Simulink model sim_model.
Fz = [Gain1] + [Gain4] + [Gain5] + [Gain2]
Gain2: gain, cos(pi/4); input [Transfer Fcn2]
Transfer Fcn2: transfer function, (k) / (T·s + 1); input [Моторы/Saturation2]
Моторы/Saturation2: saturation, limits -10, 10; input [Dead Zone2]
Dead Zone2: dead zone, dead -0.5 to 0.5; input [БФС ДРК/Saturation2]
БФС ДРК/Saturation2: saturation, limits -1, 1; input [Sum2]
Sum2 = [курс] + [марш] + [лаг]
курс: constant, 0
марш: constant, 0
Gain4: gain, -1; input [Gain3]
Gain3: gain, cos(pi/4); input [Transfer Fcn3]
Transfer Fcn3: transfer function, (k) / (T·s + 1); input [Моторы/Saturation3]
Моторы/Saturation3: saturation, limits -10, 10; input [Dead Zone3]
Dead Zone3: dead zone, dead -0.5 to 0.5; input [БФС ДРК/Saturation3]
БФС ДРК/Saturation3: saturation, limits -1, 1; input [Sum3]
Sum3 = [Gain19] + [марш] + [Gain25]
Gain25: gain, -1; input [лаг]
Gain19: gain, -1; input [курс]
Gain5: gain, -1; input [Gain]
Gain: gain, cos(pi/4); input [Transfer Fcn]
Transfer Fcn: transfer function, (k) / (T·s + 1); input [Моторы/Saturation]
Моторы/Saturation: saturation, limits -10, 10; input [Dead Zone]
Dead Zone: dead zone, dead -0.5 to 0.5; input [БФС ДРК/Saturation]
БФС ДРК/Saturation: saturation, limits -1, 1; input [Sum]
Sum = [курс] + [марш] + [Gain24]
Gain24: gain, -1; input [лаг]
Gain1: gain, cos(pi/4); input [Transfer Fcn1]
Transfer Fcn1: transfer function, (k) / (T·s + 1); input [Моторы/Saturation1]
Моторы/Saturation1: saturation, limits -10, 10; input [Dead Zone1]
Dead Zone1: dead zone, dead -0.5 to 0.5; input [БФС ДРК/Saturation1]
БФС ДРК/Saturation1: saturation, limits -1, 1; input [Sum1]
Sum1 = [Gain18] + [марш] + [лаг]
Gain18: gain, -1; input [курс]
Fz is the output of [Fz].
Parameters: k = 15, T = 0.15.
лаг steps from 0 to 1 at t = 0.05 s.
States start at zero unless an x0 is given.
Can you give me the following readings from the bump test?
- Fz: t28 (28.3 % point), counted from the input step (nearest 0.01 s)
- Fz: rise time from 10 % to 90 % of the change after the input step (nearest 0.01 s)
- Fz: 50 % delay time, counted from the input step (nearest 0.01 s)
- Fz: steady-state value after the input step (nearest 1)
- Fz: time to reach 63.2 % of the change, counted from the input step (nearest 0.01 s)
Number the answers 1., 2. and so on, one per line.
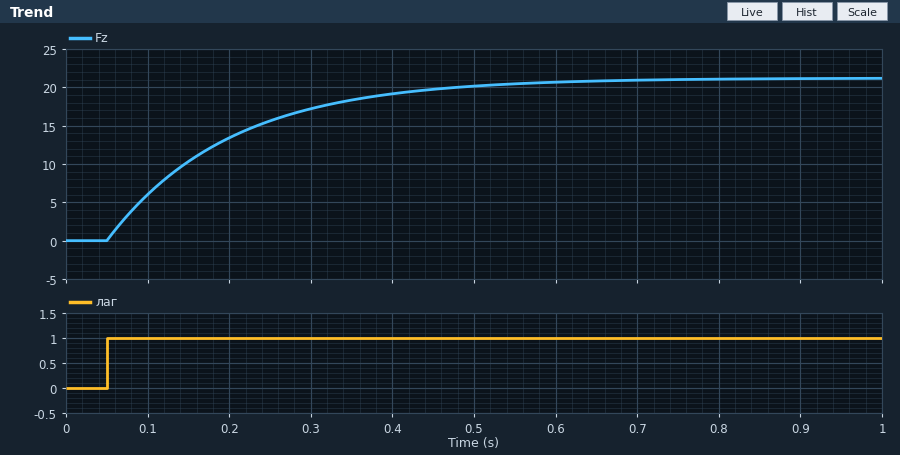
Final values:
1. 0.05 s
2. 0.33 s
3. 0.10 s
4. 21
5. 0.15 s
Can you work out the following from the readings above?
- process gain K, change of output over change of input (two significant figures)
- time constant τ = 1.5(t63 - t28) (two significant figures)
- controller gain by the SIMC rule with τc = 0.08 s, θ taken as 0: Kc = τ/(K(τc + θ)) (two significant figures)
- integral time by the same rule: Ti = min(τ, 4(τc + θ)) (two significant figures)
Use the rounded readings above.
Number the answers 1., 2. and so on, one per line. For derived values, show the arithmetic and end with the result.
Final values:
1. (21 - 0) / 1 = 21
2. 1.5 × (0.15 - 0.05) = 0.15 s
3. 0.15 / (21 × (0.08 + 0)) = 0.089
4. min(0.15, 4 × (0.08 + 0)) = 0.15 s
